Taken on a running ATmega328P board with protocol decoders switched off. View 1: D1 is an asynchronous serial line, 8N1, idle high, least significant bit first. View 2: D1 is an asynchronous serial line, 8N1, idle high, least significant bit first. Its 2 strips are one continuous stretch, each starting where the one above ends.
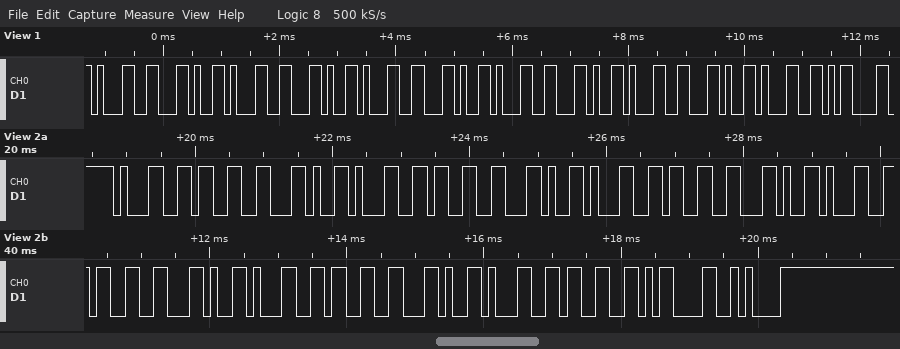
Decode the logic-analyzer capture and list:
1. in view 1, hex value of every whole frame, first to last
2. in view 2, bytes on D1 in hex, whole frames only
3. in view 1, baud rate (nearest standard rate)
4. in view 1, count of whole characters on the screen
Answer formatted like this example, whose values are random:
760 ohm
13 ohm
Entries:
0x31 0x2C 0x31 0x2C 0x31 0x2C 0x31 0x2C 0x31 0x2C 0x31 0x0D
31 33 2C 31 33 2C 31 33 2C 31 33 2C 31 33 2C 31 33 0D 0A
9600 baud
12
